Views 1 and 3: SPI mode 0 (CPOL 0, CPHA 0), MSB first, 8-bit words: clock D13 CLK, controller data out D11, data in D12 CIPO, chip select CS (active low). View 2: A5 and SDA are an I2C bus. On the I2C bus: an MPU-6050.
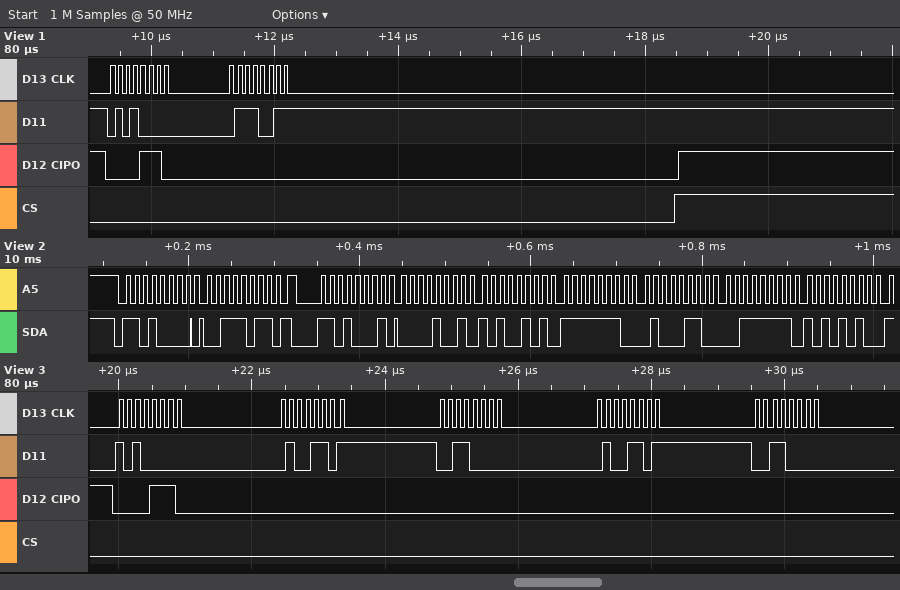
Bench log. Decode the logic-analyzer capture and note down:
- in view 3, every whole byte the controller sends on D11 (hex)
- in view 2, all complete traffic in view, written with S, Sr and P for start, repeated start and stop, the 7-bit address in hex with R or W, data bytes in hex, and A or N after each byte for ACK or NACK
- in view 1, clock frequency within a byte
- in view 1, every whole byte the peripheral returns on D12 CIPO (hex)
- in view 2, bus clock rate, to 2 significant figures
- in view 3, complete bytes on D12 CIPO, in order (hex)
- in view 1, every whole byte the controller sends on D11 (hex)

A0 4D 30 4D 30
S 68W A 3B A Sr 68R A 09 A A5 A FE A 46 A 3F A AA A
8 MHz
0E 00
100 kHz
0E 00 00 00 00
50 73
